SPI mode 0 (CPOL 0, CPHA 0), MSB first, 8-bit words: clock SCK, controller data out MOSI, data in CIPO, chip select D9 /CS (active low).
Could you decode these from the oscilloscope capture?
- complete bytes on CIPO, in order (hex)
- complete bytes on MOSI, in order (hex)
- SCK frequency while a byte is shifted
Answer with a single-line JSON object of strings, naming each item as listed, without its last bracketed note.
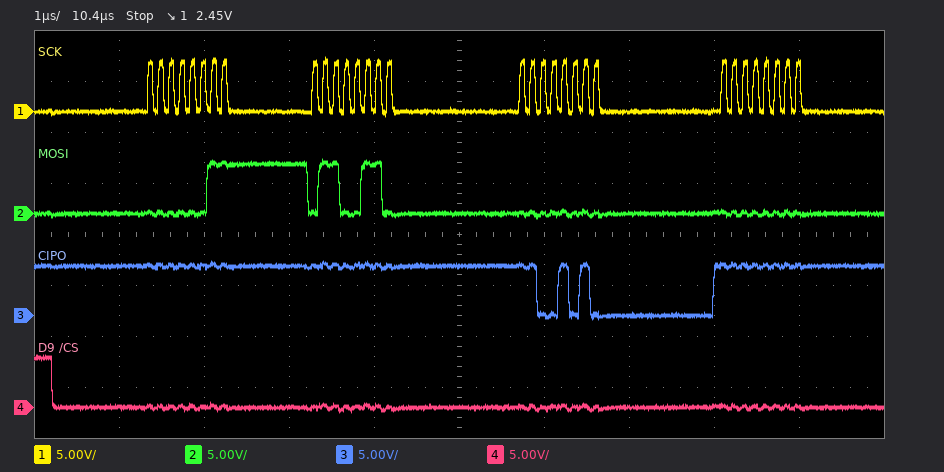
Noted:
{"complete bytes on CIPO, in order": "FF FF CA FF", "complete bytes on MOSI, in order": "03 66 00 00", "SCK frequency while a byte is shifted": "8 MHz"}
